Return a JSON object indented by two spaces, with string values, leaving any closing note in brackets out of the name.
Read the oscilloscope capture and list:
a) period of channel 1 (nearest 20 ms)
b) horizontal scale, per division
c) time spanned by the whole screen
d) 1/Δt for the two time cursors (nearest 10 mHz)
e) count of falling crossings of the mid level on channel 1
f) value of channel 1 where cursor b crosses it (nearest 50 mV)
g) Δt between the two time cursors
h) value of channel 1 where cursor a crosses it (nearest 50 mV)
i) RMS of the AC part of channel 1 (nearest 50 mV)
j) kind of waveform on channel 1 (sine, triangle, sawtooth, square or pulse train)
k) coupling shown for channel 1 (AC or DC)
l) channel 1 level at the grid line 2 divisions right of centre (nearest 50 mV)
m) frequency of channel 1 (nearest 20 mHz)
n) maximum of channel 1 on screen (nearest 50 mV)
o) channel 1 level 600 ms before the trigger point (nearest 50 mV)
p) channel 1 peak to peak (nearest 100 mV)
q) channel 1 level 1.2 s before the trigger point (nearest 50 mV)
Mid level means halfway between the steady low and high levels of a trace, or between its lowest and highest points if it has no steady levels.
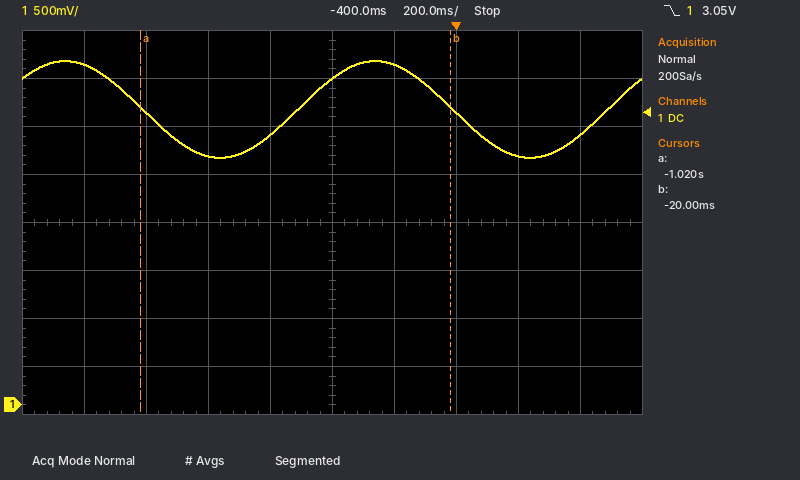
{
  "period of channel 1": "1.00 s",
  "horizontal scale, per division": "200 ms",
  "time spanned by the whole screen": "2 s",
  "1/Δt for the two time cursors": "1.00 Hz",
  "count of falling crossings of the mid level on channel 1": "2",
  "value of channel 1 where cursor b crosses it": "3.10 V",
  "Δt between the two time cursors": "1.00 s",
  "value of channel 1 where cursor a crosses it": "3.10 V",
  "RMS of the AC part of channel 1": "350 mV",
  "kind of waveform on channel 1": "sine",
  "coupling shown for channel 1": "DC",
  "channel 1 level at the grid line 2 divisions right of centre": "3.05 V",
  "frequency of channel 1": "1.00 Hz",
  "maximum of channel 1 on screen": "3.60 V",
  "channel 1 level 600 ms before the trigger point": "2.80 V",
  "channel 1 peak to peak": "1.00 V",
  "channel 1 level 1.2 s before the trigger point": "3.55 V"
}
